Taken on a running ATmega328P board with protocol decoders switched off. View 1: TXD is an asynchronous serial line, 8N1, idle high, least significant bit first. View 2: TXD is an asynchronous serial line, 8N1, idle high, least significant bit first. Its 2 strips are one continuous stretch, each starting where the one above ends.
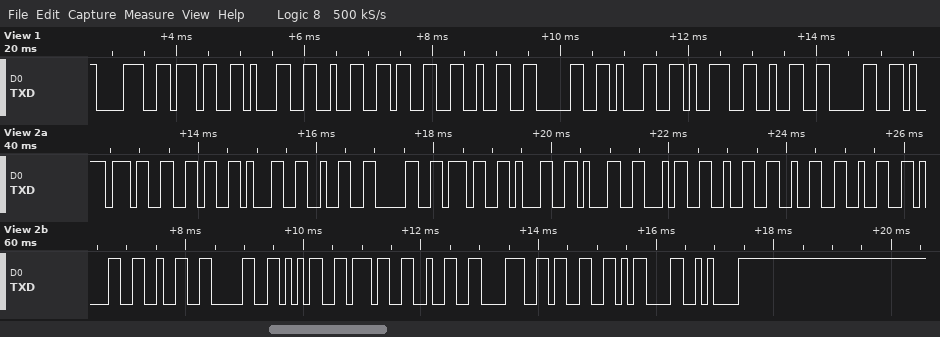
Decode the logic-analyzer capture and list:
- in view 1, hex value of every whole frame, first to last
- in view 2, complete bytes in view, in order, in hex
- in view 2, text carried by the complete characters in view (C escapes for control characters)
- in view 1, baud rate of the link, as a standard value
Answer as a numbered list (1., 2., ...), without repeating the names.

1. 38 37 31 32 33 32 30 31 39 32 30
2. 0x37 0x36 0x31 0x32 0x30 0x37 0x31 0x31 0x34 0x32 0x32 0x32 0x31 0x32 0x30 0x35 0x37 0x32 0x38 0x33 0x0D 0x0A
3. "76120711422212057283\r\n"
4. 9600 baud
